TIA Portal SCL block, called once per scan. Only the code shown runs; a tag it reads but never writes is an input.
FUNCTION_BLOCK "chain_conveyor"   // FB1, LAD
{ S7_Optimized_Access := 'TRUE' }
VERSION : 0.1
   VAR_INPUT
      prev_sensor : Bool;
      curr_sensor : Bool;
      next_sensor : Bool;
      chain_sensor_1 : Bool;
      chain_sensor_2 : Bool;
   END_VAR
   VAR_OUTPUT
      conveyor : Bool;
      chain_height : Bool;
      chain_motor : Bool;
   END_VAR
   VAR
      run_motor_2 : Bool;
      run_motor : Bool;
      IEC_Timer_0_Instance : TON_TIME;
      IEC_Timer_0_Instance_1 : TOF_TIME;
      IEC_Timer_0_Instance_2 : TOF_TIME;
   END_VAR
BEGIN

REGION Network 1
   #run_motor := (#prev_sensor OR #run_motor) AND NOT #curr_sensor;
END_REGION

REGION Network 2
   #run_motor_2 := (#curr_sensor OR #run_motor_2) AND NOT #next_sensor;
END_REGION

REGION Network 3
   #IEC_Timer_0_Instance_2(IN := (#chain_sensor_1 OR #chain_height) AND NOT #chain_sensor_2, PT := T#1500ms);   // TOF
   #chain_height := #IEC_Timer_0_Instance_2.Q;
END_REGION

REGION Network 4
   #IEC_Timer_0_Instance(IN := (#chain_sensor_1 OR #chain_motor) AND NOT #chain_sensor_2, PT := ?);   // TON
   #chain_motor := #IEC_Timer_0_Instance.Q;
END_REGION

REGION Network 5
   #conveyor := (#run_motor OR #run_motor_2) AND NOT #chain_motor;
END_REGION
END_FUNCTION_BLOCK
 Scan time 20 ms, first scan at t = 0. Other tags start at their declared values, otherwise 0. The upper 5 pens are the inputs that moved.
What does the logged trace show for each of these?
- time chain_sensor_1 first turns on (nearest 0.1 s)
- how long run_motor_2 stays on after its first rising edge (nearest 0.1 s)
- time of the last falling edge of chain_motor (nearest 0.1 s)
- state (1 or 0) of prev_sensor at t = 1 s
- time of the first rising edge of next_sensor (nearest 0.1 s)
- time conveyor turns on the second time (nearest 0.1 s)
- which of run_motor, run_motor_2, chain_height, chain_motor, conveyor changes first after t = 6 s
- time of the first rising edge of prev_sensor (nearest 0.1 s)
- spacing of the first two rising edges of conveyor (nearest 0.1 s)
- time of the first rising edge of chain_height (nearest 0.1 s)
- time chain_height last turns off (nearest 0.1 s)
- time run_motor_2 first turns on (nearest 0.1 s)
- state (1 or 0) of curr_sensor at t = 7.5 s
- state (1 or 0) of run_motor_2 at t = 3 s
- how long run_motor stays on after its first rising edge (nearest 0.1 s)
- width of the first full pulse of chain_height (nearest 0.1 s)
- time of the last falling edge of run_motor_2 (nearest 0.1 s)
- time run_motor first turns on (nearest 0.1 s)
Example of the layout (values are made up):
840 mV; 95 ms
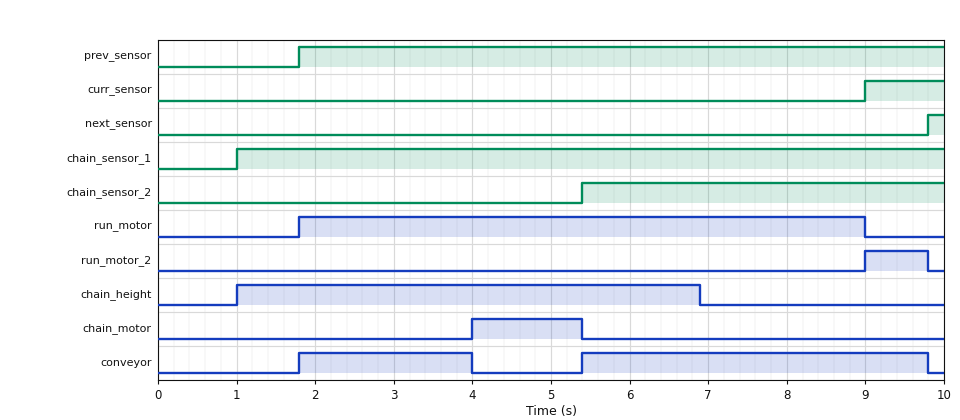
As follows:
1.0 s; 0.8 s; 5.4 s; 0; 9.8 s; 5.4 s; chain_height; 1.8 s; 3.6 s; 1.0 s; 6.9 s; 9.0 s; 0; 0; 7.2 s; 5.9 s; 9.8 s; 1.8 s
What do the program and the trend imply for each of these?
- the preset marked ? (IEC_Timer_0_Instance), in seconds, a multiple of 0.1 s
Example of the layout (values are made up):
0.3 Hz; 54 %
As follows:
3.0 s
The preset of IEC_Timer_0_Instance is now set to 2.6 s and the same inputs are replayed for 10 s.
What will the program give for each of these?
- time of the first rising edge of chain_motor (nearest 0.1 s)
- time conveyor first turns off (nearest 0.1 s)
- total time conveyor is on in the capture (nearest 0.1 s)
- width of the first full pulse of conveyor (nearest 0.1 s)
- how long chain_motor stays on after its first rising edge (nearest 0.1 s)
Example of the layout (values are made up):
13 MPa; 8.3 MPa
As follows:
3.6 s; 3.6 s; 6.2 s; 1.8 s; 1.8 s
